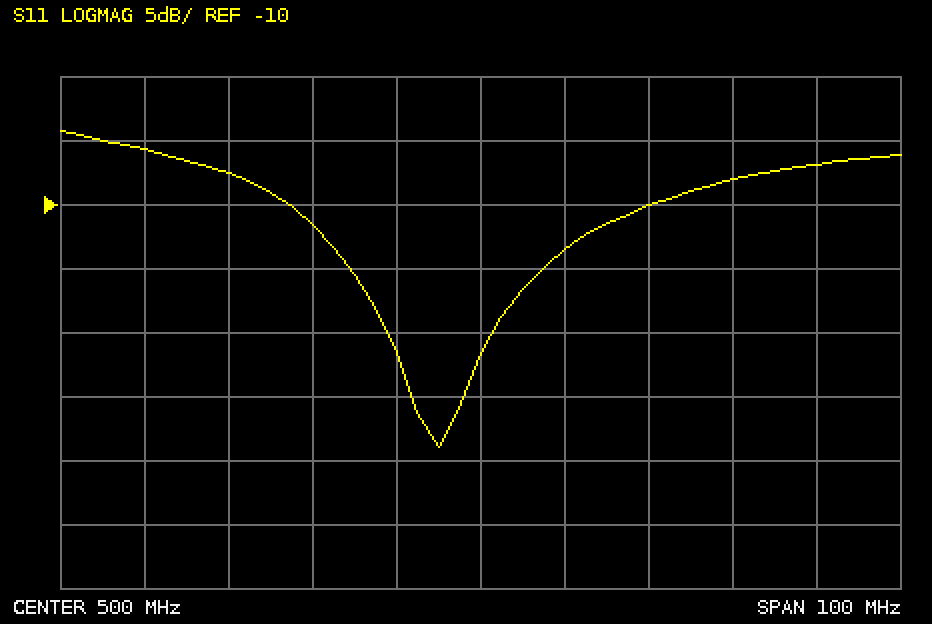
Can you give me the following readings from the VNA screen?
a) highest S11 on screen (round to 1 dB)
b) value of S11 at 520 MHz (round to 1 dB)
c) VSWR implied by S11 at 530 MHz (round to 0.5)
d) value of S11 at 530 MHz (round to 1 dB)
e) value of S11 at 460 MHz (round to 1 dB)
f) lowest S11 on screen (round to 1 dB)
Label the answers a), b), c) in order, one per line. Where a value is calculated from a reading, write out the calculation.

a) -4 dB
b) -10 dB
c) |Γ| = 10^(-8/20) = 0.3981; VSWR = (1 + 0.3981)/(1 − 0.3981) ≈ 2.32, so 2.5 to the nearest 0.5
d) -8 dB
e) -6 dB
f) -29 dB
